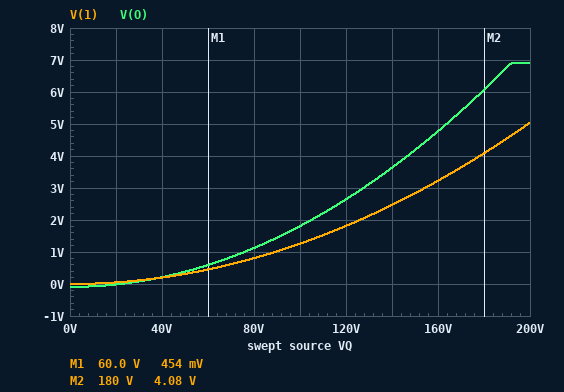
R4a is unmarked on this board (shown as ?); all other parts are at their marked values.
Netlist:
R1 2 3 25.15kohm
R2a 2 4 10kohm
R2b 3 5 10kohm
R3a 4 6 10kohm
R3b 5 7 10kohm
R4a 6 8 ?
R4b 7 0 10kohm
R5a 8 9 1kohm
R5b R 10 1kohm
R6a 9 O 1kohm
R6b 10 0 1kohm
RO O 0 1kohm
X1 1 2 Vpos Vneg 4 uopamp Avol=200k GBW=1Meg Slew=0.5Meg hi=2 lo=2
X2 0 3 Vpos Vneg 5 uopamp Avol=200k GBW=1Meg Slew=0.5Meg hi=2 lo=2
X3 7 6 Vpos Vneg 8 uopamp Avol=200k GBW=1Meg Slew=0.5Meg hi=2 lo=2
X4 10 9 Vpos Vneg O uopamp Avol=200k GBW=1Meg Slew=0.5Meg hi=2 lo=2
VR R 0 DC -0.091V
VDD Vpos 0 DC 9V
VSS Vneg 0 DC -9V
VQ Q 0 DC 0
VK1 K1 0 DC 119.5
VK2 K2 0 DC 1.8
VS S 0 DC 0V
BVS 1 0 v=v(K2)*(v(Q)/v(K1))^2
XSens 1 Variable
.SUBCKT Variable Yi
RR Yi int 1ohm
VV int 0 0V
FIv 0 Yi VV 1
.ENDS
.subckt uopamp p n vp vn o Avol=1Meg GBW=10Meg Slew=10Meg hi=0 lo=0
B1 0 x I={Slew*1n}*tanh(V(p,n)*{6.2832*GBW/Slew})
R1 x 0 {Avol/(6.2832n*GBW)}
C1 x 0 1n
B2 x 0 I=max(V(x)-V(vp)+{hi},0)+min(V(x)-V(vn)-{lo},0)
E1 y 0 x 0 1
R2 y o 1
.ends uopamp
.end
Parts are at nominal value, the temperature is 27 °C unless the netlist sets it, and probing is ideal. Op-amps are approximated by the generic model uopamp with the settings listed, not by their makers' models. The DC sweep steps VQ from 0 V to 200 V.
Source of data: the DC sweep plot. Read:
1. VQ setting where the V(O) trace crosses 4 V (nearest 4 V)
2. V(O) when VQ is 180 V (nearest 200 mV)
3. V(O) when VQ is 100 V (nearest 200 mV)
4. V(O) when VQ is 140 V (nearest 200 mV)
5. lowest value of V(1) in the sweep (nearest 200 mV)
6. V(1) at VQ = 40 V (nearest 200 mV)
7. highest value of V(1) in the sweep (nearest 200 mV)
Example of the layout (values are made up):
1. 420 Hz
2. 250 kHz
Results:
1. 148 V
2. 6.0 V
3. 1.8 V
4. 3.6 V
5. 0 V
6. 200 mV
7. 5.0 V
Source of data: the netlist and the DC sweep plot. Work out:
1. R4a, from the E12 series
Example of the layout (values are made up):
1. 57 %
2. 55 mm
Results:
1. 8.2 kΩ
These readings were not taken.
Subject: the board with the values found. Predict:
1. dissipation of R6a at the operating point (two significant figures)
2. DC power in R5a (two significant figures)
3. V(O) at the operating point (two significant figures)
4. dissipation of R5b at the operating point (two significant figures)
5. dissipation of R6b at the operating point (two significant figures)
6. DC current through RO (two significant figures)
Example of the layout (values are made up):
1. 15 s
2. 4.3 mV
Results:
1. 2.1 µW
2. 2.1 µW
3. -91 mV
4. 2.1 µW
5. 2.1 µW
6. 91 µA
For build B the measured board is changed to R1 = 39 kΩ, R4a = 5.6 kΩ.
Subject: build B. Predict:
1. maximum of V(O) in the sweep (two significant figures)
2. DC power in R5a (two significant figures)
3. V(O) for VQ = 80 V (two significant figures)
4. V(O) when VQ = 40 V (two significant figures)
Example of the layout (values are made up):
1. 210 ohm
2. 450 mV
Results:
1. 4.5 V
2. 2.1 µW
3. 640 mV
4. 91 mV
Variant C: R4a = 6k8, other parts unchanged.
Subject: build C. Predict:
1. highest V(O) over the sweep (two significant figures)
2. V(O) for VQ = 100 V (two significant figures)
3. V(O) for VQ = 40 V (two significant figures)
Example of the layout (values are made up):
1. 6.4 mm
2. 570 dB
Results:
1. 6.3 V
2. 1.5 V
3. 170 mV
